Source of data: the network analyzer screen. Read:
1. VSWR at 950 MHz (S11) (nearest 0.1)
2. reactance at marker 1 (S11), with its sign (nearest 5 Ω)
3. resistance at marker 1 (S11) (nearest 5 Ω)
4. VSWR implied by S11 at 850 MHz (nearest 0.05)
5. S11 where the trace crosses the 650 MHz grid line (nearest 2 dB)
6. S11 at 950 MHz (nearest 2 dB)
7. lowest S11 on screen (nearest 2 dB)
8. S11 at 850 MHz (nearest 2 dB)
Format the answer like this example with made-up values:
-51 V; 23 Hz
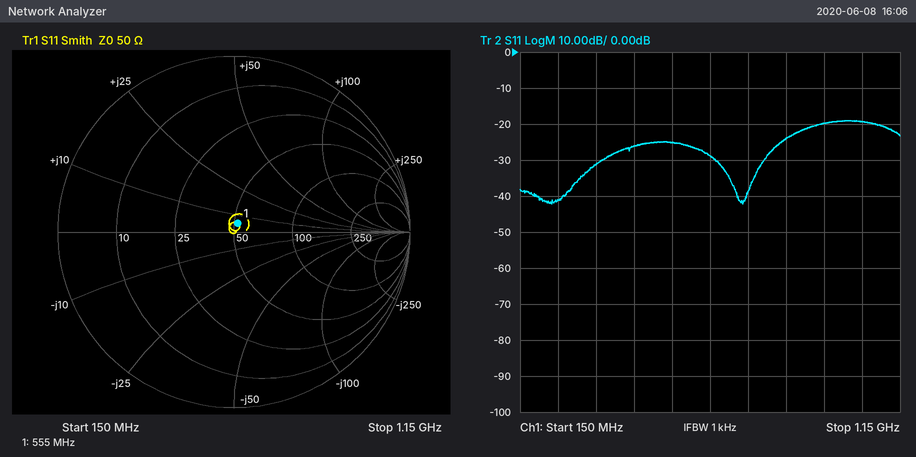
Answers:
1.2; +5 Ω; 50 Ω; 1.15; -28 dB; -20 dB; -42 dB; -24 dB
